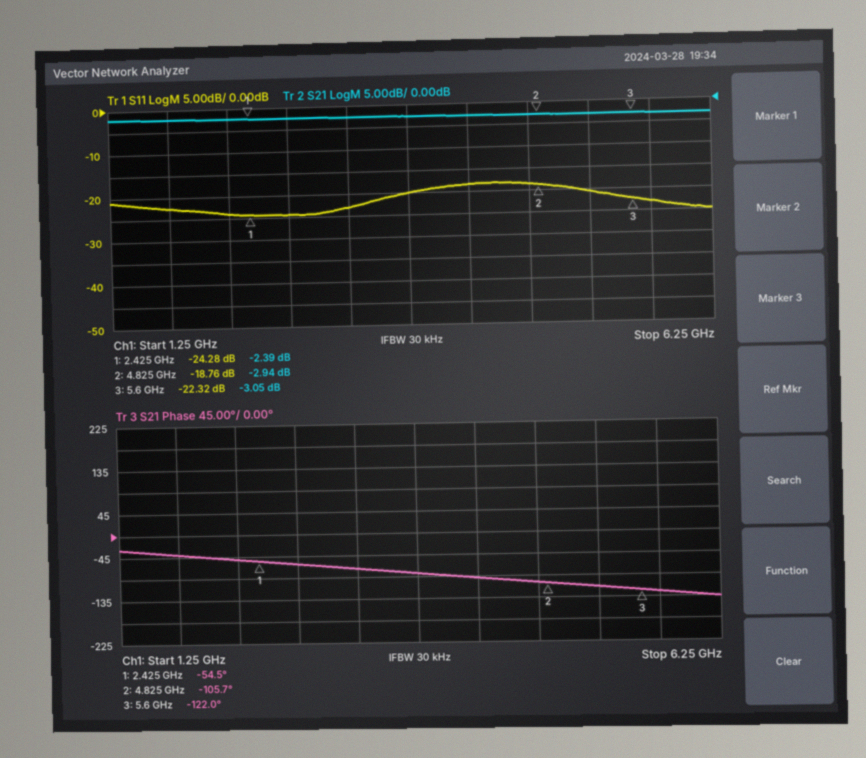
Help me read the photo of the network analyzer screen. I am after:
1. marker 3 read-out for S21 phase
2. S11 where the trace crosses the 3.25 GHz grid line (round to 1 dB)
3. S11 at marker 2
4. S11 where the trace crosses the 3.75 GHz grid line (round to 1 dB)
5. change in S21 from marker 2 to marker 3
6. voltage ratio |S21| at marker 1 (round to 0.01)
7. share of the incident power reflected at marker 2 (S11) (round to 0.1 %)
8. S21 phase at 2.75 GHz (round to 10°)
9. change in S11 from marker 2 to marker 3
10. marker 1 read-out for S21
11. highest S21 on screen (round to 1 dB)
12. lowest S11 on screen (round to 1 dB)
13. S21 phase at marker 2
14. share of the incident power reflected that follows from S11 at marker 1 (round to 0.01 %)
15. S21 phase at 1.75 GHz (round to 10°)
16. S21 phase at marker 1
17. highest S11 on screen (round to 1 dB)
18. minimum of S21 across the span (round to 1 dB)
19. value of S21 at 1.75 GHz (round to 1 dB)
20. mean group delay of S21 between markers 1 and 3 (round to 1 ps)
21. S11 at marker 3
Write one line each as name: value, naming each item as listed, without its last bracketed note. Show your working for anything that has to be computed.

marker 3 read-out for S21 phase: -122.0°
S11 where the trace crosses the 3.25 GHz grid line: -23 dB
S11 at marker 2: -18.76 dB
S11 where the trace crosses the 3.75 GHz grid line: -20 dB
change in S21 from marker 2 to marker 3: -3.05 − (-2.94) = -0.11 dB
voltage ratio |S21| at marker 1: 10^(-2.39/20) ≈ 0.76
share of the incident power reflected at marker 2 (S11): 10^(-18.76/10) ≈ 1.3 %
S21 phase at 2.75 GHz: -60°
change in S11 from marker 2 to marker 3: -22.32 − (-18.76) = -3.56 dB
marker 1 read-out for S21: -2.39 dB
highest S21 on screen: -2 dB
lowest S11 on screen: -25 dB
S21 phase at marker 2: -105.7°
share of the incident power reflected that follows from S11 at marker 1: 10^(-24.28/10) ≈ 0.37 %
S21 phase at 1.75 GHz: -40°
S21 phase at marker 1: -54.5°
highest S11 on screen: -18 dB
minimum of S21 across the span: -3 dB
value of S21 at 1.75 GHz: -2 dB
mean group delay of S21 between markers 1 and 3: −(-122° − (-54.5°))/(360° × 3.175 GHz) ≈ 59 ps
S11 at marker 3: -22.32 dB
